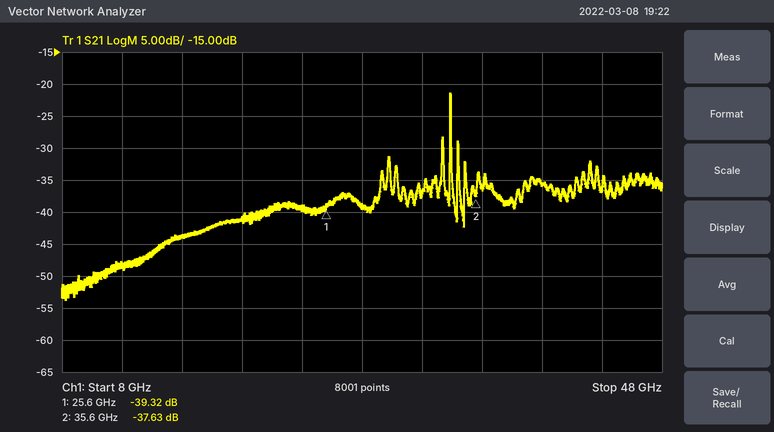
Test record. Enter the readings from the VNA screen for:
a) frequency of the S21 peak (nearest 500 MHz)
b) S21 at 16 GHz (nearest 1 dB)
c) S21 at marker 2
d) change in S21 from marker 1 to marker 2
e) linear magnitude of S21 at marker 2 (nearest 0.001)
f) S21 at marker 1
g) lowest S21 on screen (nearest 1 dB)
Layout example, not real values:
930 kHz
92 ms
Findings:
34.0 GHz
-44 dB
-37.63 dB
1.69 dB
0.013
-39.32 dB
-54 dB
